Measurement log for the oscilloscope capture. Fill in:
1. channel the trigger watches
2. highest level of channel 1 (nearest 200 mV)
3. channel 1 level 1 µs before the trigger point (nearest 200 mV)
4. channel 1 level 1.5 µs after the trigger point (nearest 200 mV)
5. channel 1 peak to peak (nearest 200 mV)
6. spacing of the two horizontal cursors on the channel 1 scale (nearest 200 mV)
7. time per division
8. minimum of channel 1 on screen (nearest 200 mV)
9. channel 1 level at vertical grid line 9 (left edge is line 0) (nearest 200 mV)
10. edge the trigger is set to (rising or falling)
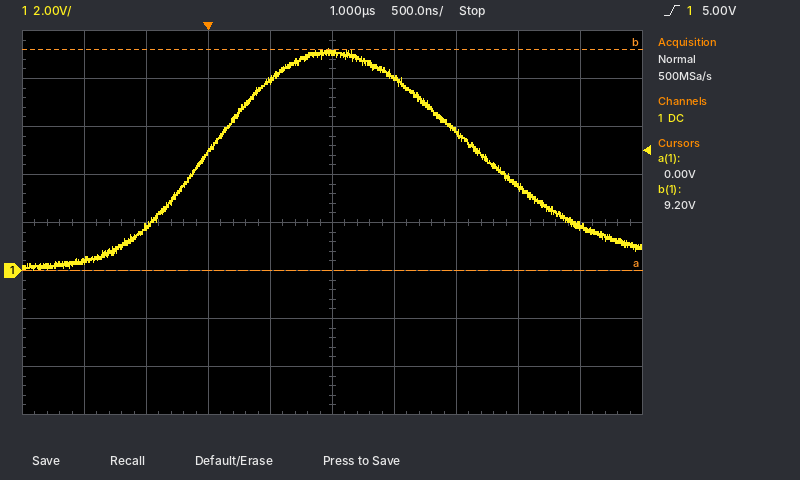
channel 1
9.2 V
400 mV
8.0 V
9.2 V
9.2 V
500 ns
0.0 V
1.8 V
rising
